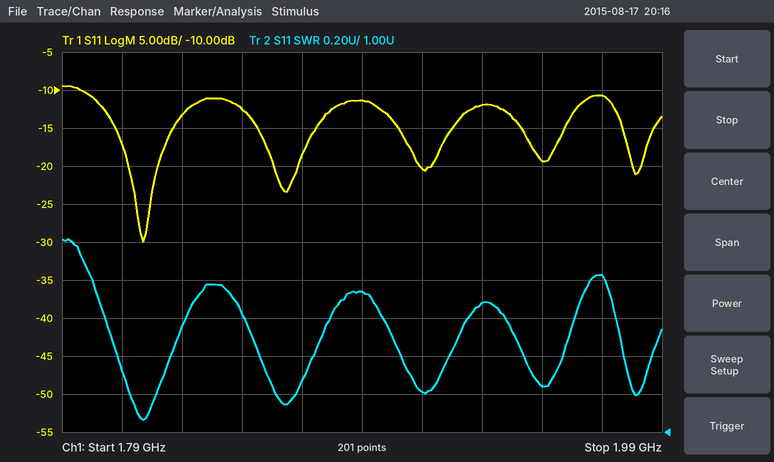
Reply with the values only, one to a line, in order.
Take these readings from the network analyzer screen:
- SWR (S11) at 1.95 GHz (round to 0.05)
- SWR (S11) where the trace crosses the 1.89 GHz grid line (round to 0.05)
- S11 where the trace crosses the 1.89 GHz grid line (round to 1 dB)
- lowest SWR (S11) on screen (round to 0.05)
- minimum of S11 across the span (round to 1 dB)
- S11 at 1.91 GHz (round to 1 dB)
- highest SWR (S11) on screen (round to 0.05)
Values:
1.25
1.75
-11 dB
1.05
-30 dB
-20 dB
2.00
